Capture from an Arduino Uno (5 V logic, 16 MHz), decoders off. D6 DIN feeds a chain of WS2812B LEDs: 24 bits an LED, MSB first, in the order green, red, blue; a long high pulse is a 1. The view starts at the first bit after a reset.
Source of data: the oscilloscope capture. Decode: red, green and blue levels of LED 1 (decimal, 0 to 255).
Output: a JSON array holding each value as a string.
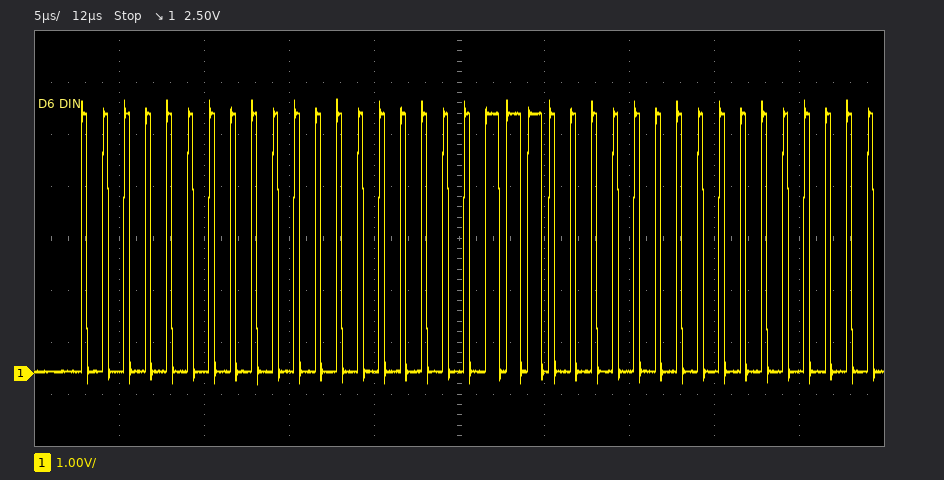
["0, 0, 28"]
